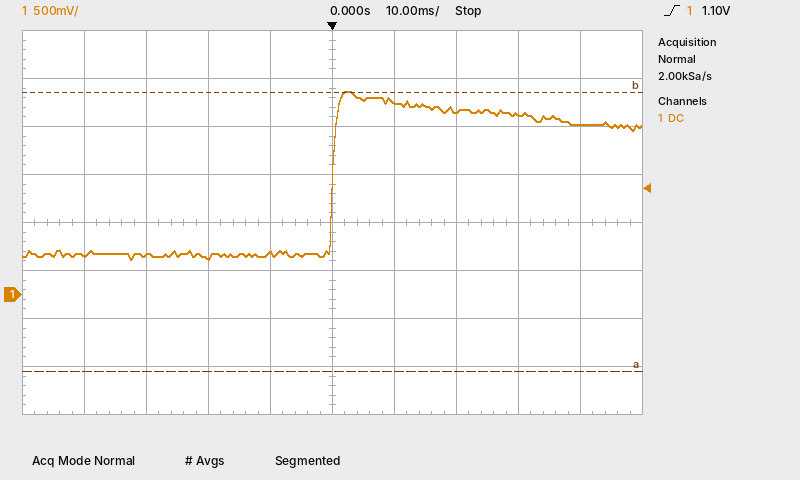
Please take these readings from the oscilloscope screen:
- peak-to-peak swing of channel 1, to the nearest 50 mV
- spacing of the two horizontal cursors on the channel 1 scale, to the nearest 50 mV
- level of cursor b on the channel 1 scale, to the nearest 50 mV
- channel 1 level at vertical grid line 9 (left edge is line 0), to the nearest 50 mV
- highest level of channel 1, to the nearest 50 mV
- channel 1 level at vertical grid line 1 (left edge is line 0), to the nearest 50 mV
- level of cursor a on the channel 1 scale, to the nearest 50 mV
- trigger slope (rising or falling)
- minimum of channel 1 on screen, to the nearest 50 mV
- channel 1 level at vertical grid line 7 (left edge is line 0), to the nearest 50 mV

1.75 V
2.90 V
2.10 V
1.75 V
2.10 V
400 mV
-800 mV
rising
350 mV
1.90 V
